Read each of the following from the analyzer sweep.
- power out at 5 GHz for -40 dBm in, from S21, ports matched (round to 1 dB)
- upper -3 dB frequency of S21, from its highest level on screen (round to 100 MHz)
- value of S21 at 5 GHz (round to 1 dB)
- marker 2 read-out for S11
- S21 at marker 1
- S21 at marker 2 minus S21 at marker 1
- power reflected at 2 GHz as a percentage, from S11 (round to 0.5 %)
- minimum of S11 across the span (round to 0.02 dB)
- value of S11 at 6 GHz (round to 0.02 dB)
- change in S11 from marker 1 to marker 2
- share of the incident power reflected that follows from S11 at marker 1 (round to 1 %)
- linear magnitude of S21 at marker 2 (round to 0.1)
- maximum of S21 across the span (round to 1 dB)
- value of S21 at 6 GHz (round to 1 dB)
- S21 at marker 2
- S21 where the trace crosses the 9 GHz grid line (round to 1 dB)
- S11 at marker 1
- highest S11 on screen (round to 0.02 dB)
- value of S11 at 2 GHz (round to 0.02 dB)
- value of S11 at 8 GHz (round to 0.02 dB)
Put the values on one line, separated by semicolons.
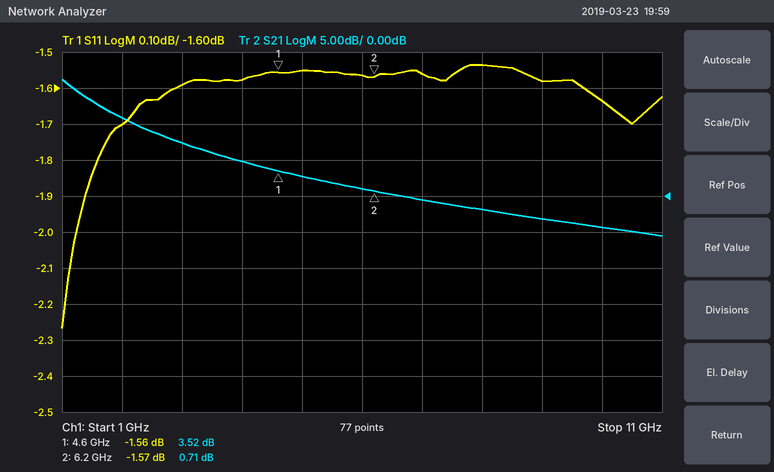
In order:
-37 dBm; 1.5 GHz; 3 dB; -1.57 dB; 3.52 dB; -2.81 dB; 67.5 %; -2.26 dB; -1.56 dB; -0.01 dB; 70 %; 1.1; 16 dB; 1 dB; 0.71 dB; -3 dB; -1.56 dB; -1.54 dB; -1.70 dB; -1.54 dB
